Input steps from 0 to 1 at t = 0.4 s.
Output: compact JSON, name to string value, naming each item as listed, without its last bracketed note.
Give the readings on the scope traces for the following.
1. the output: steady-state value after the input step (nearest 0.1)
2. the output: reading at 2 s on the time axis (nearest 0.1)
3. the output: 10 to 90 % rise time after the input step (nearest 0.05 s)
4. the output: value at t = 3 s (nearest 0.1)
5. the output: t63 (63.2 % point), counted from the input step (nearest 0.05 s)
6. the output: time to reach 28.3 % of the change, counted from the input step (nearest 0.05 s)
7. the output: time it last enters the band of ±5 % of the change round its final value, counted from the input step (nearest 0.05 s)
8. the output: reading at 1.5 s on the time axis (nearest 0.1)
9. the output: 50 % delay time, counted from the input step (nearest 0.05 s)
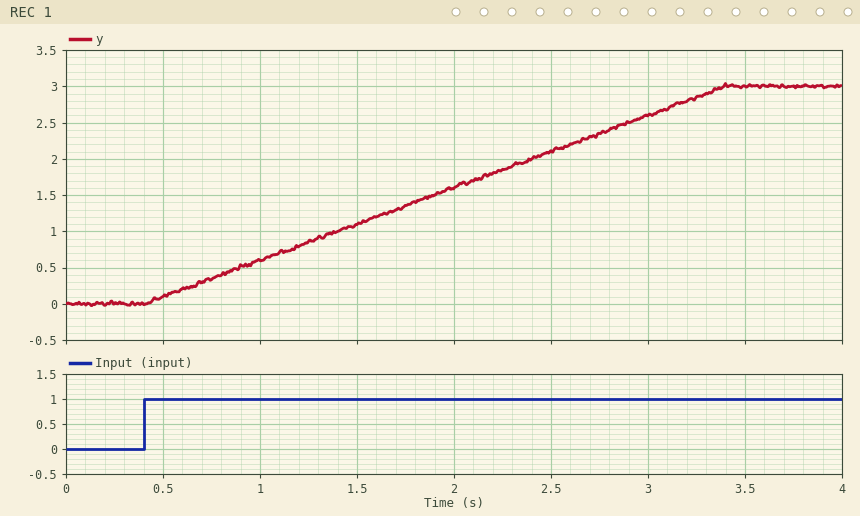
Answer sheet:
{"the output: steady-state value after the input step": "3.0", "the output: reading at 2 s on the time axis": "1.6", "the output: 10 to 90 % rise time after the input step": "2.40 s", "the output: value at t = 3 s": "2.6", "the output: t63 (63.2 % point), counted from the input step": "1.90 s", "the output: time to reach 28.3 % of the change, counted from the input step": "0.85 s", "the output: time it last enters the band of ±5 % of the change round its final value, counted from the input step": "2.85 s", "the output: reading at 1.5 s on the time axis": "1.1", "the output: 50 % delay time, counted from the input step": "1.50 s"}
